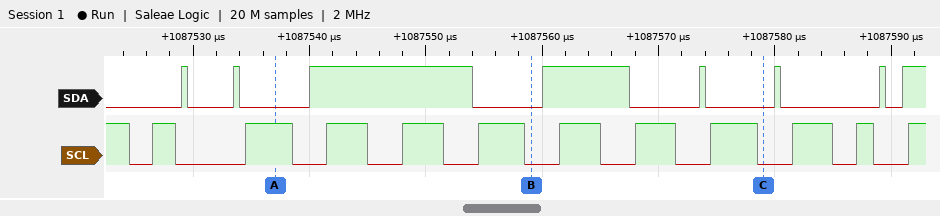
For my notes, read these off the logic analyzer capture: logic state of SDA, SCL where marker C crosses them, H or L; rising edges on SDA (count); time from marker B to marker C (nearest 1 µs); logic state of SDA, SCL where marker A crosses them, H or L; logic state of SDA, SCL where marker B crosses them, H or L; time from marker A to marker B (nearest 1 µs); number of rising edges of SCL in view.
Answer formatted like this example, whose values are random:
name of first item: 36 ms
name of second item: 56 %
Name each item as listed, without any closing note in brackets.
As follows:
logic state of SDA, SCL where marker C crosses them, H or L: SDA=L, SCL=L
rising edges on SDA: 8
time from marker B to marker C: 20 µs
logic state of SDA, SCL where marker A crosses them, H or L: SDA=L, SCL=H
logic state of SDA, SCL where marker B crosses them, H or L: SDA=L, SCL=L
time from marker A to marker B: 22 µs
number of rising edges of SCL in view: 11
